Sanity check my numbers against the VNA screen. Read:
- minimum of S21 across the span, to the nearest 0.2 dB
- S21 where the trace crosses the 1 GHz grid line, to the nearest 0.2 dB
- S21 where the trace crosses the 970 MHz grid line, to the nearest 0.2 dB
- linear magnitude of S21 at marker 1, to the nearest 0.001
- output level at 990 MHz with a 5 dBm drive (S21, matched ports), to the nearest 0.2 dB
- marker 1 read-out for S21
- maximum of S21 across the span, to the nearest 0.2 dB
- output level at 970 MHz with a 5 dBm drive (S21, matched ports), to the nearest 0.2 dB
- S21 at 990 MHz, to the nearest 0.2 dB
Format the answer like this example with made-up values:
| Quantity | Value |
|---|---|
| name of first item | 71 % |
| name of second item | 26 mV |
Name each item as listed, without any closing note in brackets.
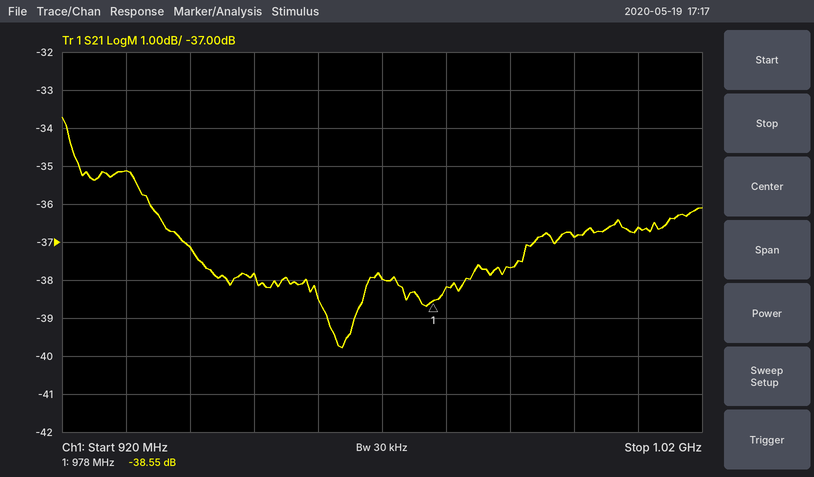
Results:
| Quantity | Value |
|---|---|
| minimum of S21 across the span, to the nearest 0.2 dB | -39.8 dB |
| S21 where the trace crosses the 1 GHz grid line, to the nearest 0.2 dB | -36.8 dB |
| S21 where the trace crosses the 970 MHz grid line, to the nearest 0.2 dB | -38.0 dB |
| linear magnitude of S21 at marker 1, to the nearest 0.001 | 0.012 |
| output level at 990 MHz with a 5 dBm drive (S21, matched ports), to the nearest 0.2 dB | -32.6 dBm |
| marker 1 read-out for S21 | -38.55 dB |
| maximum of S21 across the span, to the nearest 0.2 dB | -33.8 dB |
| output level at 970 MHz with a 5 dBm drive (S21, matched ports), to the nearest 0.2 dB | -33.0 dBm |
| S21 at 990 MHz, to the nearest 0.2 dB | -37.6 dB |
